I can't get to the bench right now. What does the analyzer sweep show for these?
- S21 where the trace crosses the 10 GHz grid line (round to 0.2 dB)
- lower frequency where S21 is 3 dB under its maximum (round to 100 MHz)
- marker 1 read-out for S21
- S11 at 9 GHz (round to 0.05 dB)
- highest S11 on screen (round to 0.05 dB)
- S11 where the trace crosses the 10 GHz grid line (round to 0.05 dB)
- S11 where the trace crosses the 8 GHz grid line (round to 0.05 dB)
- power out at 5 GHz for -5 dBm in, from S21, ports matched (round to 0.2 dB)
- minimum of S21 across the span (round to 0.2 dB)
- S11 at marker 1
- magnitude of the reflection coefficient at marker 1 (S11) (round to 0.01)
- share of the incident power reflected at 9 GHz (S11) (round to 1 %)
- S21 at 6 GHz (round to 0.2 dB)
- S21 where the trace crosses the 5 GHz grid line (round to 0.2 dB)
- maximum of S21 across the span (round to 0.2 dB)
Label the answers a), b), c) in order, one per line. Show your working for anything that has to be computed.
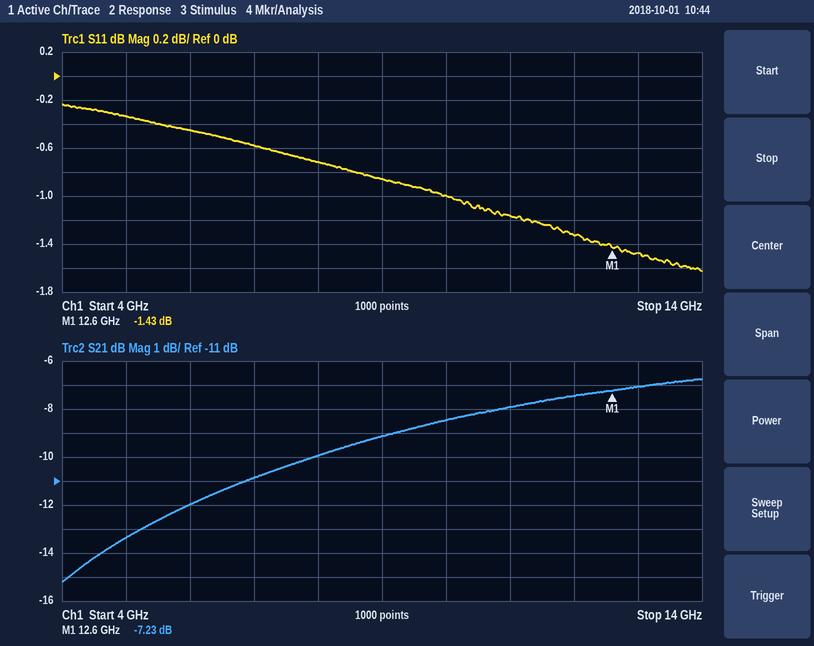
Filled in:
a) -8.4 dB
b) 8.2 GHz
c) -7.23 dB
d) -0.85 dB
e) -0.25 dB
f) -1.00 dB
g) -0.70 dB
h) -5 dBm + (-13.4 dB) = -18.4 dBm
i) -15.2 dB
j) -1.43 dB
k) 10^(-1.43/20) ≈ 0.85
l) 10^(-0.85/10) ≈ 82 %
m) -12.0 dB
n) -13.4 dB
o) -6.8 dB
